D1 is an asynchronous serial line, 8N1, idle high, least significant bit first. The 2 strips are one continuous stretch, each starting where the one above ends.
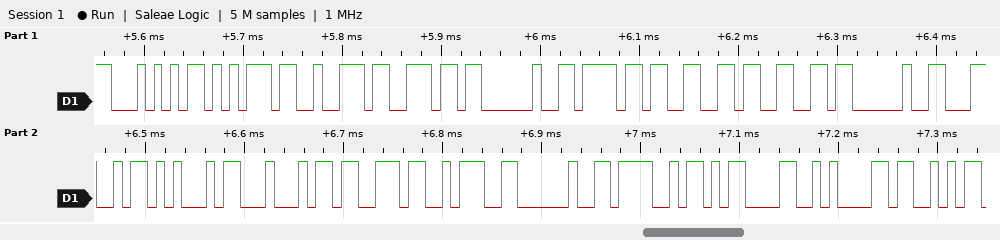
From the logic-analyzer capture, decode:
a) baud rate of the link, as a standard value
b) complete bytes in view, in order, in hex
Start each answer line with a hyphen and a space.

- 115200 baud
- 0x54 0x75 0x72 0x6E 0x20 0x6F 0x66 0x66 0x20 0x4C 0x45 0x44 0x73 0x3A 0x20 0x4F 0x0D 0x0A 0x53
